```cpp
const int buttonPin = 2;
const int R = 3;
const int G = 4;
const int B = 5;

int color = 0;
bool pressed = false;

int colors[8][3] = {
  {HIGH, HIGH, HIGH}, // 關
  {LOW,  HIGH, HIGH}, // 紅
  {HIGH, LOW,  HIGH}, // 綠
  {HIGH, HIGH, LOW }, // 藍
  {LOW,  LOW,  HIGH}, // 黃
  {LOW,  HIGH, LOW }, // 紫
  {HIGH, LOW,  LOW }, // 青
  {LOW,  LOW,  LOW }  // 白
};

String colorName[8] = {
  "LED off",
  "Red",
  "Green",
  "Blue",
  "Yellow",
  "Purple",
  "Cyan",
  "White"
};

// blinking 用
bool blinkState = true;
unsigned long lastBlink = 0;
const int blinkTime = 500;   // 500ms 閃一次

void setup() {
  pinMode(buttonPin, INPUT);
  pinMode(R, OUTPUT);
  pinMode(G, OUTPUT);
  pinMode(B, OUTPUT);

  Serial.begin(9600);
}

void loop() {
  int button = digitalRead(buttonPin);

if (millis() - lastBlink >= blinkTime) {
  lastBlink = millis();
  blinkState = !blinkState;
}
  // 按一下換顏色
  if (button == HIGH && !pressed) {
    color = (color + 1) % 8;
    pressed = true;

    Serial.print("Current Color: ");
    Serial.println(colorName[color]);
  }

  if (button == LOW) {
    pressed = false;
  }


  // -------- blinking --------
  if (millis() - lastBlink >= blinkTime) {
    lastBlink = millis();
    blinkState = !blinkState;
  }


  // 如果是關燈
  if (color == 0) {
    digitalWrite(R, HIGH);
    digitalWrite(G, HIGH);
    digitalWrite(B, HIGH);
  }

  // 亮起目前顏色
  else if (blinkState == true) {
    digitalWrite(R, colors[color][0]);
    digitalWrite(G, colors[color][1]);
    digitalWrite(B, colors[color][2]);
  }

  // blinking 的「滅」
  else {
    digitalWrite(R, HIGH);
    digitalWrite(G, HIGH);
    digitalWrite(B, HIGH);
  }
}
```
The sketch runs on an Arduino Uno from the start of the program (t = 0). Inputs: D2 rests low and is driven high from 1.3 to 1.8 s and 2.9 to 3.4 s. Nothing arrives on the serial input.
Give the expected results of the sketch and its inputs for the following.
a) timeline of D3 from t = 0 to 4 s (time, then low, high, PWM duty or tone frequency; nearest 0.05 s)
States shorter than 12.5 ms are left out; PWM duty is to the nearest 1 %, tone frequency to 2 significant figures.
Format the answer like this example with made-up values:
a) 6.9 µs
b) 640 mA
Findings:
a) 0 s high; 1.3 s low; 1.5 s high; 2 s low; 2.5 s high
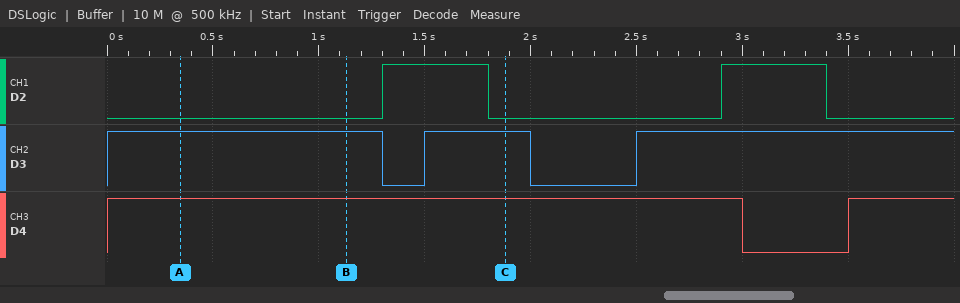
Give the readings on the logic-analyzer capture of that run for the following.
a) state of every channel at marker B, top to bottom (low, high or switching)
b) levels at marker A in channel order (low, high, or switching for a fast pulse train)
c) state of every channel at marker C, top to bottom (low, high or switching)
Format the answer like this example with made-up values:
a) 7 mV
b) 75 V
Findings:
a) D2 low, D3 high, D4 high
b) D2 low, D3 high, D4 high
c) D2 low, D3 high, D4 high
